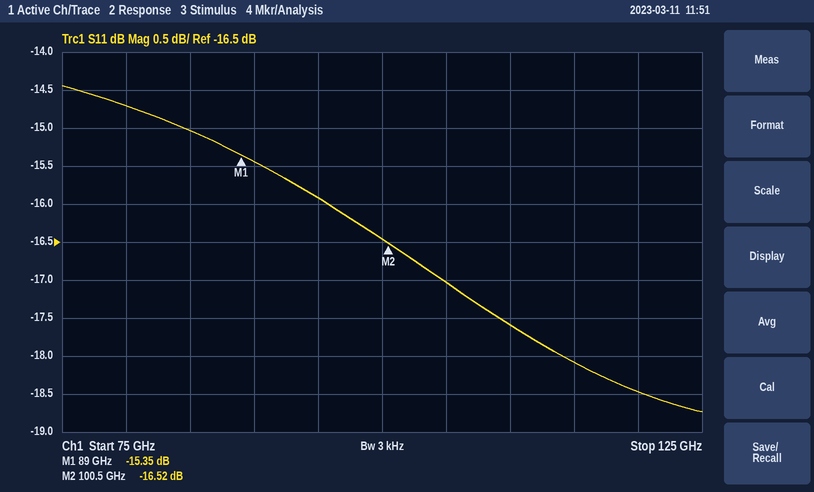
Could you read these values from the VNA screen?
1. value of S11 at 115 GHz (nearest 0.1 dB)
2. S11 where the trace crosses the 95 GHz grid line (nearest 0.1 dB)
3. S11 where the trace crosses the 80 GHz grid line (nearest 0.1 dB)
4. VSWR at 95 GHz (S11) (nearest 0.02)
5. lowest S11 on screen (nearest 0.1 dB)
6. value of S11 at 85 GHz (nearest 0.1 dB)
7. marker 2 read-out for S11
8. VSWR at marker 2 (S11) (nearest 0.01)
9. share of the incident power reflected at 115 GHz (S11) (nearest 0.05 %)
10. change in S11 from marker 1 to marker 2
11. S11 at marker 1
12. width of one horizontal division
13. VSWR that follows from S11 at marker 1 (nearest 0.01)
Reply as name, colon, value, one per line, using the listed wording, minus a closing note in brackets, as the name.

value of S11 at 115 GHz: -18.1 dB
S11 where the trace crosses the 95 GHz grid line: -15.9 dB
S11 where the trace crosses the 80 GHz grid line: -14.7 dB
VSWR at 95 GHz (S11): 1.38
lowest S11 on screen: -18.7 dB
value of S11 at 85 GHz: -15.0 dB
marker 2 read-out for S11: -16.52 dB
VSWR at marker 2 (S11): 1.35
share of the incident power reflected at 115 GHz (S11): 1.55 %
change in S11 from marker 1 to marker 2: -1.17 dB
S11 at marker 1: -15.35 dB
width of one horizontal division: 5 GHz
VSWR that follows from S11 at marker 1: 1.41
